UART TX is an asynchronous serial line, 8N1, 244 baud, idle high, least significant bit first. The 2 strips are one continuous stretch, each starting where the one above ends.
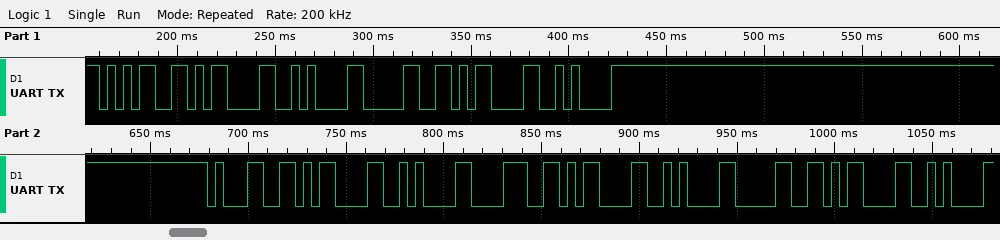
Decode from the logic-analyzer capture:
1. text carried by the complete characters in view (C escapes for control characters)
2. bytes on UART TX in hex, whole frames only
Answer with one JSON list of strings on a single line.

["\"5\\r\\n0\\r\\n1\\r\\n8\\r\\n0\\r\\n\"", "0x35 0x0D 0x0A 0x30 0x0D 0x0A 0x31 0x0D 0x0A 0x38 0x0D 0x0A 0x30 0x0D 0x0A"]
